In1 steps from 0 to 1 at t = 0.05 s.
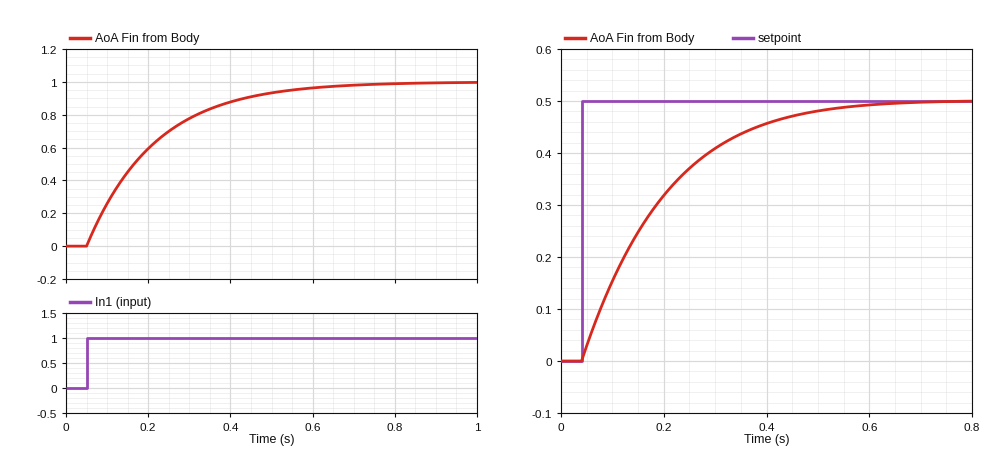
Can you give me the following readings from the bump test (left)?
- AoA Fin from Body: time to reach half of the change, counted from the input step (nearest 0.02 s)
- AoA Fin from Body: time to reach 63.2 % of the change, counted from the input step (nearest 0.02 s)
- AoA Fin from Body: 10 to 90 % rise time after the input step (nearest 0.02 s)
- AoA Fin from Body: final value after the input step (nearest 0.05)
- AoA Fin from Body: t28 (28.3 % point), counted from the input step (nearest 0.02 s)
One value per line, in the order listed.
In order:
0.12 s
0.16 s
0.36 s
1.00
0.06 s
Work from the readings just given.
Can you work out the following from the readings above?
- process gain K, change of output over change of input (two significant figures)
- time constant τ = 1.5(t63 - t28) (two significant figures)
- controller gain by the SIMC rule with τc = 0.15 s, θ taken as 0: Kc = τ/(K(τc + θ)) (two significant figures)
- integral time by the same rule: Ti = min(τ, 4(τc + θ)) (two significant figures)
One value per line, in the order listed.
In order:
1.0
0.15 s
1.0
0.15 s
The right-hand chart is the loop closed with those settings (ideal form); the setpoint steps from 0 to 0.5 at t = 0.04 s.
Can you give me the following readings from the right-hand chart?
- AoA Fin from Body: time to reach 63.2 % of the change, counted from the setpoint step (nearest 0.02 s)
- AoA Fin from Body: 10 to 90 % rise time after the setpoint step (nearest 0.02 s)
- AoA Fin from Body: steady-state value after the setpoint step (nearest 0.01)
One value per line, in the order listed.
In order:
0.16 s
0.32 s
0.50
